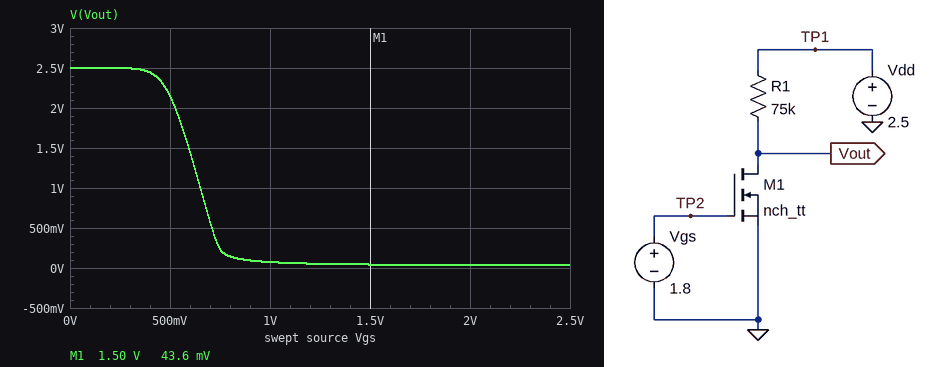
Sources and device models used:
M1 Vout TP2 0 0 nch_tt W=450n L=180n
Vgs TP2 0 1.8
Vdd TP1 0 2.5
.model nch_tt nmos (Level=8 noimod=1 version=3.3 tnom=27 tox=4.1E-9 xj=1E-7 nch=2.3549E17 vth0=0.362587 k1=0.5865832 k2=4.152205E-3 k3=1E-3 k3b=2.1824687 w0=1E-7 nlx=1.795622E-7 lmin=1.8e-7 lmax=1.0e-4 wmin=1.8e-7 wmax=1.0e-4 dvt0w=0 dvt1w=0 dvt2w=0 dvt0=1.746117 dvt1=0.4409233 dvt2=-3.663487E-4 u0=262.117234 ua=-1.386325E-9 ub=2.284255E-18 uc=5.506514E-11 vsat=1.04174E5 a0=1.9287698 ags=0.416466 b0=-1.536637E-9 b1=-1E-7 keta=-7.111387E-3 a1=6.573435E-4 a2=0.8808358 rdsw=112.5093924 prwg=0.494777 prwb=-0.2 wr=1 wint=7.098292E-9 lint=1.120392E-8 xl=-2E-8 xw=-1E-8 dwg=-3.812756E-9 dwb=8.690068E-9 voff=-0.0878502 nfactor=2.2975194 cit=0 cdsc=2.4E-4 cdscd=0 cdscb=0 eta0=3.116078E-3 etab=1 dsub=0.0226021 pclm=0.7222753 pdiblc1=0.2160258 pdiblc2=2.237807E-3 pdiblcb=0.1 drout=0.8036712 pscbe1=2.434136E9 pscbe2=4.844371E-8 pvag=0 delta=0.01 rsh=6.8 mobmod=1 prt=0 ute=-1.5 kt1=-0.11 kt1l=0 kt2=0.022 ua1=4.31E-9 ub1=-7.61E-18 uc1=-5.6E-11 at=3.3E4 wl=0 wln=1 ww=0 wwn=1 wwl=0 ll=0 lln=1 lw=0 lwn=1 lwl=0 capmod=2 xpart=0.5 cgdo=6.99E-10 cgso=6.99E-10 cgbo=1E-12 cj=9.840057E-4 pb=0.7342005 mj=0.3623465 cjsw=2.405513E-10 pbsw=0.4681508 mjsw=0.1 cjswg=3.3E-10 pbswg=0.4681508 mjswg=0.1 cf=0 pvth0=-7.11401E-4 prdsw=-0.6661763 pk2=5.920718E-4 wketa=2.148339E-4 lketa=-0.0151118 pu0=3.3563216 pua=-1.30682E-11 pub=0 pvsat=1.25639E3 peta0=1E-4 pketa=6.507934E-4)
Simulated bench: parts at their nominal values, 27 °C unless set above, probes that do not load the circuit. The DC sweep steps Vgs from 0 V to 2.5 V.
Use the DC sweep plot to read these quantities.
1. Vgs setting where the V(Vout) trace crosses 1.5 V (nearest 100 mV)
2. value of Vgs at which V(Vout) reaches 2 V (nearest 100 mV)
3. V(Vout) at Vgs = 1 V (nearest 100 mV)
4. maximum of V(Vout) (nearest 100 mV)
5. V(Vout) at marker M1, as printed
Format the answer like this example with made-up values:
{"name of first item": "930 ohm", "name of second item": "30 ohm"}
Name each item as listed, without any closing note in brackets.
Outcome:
{"Vgs setting where the V(Vout) trace crosses 1.5 V": "600 mV", "value of Vgs at which V(Vout) reaches 2 V": "500 mV", "V(Vout) at Vgs = 1 V": "100 mV", "maximum of V(Vout)": "2.5 V", "V(Vout) at marker M1, as printed": "43.6 mV"}
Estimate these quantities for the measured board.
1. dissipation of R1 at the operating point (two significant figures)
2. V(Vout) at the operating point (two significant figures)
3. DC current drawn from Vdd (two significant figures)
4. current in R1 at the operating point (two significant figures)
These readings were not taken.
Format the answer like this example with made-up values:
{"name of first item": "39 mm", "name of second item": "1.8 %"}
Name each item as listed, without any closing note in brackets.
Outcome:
{"dissipation of R1 at the operating point": "81 µW", "V(Vout) at the operating point": "39 mV", "DC current drawn from Vdd": "33 µA", "current in R1 at the operating point": "33 µA"}
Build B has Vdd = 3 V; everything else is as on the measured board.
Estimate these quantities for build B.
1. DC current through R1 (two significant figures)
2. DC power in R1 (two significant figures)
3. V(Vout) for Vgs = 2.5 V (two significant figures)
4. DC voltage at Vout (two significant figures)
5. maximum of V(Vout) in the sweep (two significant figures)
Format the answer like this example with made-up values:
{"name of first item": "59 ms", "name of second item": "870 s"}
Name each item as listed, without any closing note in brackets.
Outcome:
{"DC current through R1": "39 µA", "DC power in R1": "120 µW", "V(Vout) for Vgs = 2.5 V": "44 mV", "DC voltage at Vout": "47 mV", "maximum of V(Vout) in the sweep": "3.0 V"}
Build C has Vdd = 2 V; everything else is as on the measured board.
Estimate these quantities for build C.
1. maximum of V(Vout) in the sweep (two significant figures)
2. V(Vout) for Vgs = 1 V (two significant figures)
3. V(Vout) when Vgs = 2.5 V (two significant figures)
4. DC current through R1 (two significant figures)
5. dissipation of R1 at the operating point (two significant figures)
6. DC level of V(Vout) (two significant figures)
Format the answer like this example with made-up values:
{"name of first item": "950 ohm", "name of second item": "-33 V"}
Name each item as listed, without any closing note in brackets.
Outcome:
{"maximum of V(Vout) in the sweep": "2.0 V", "V(Vout) for Vgs = 1 V": "58 mV", "V(Vout) when Vgs = 2.5 V": "29 mV", "DC current through R1": "26 µA", "dissipation of R1 at the operating point": "52 µW", "DC level of V(Vout)": "31 mV"}
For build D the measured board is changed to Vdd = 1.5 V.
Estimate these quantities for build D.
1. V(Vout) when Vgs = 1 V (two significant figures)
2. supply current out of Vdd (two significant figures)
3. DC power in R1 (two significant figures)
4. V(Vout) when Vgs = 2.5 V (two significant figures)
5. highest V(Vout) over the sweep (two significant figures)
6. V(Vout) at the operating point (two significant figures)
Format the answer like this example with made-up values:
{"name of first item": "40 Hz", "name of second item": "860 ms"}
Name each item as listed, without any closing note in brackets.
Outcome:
{"V(Vout) when Vgs = 1 V": "42 mV", "supply current out of Vdd": "20 µA", "DC power in R1": "29 µW", "V(Vout) when Vgs = 2.5 V": "22 mV", "highest V(Vout) over the sweep": "1.5 V", "V(Vout) at the operating point": "23 mV"}
